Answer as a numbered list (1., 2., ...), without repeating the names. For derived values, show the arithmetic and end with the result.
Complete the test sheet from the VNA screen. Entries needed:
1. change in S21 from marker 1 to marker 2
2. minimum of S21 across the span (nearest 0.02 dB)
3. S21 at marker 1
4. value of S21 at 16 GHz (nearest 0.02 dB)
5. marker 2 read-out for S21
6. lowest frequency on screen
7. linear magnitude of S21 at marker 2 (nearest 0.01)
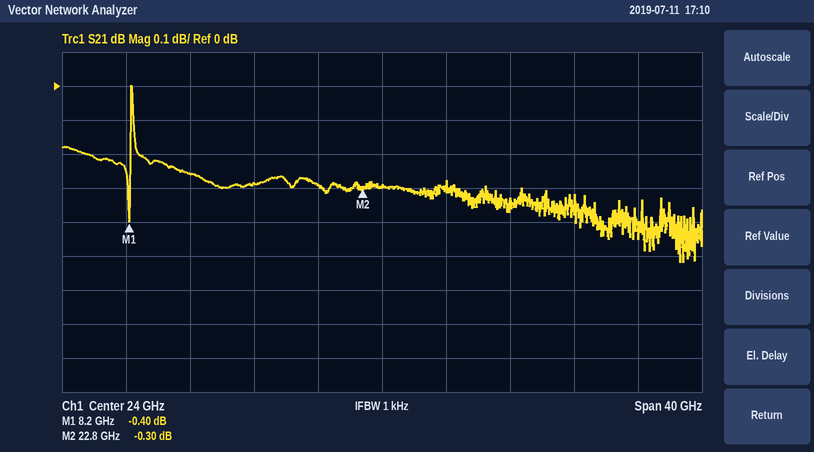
1. -0.3 − (-0.4) = 0.10 dB
2. -0.52 dB
3. -0.40 dB
4. -0.28 dB
5. -0.30 dB
6. 4 GHz
7. 10^(-0.3/20) ≈ 0.97
